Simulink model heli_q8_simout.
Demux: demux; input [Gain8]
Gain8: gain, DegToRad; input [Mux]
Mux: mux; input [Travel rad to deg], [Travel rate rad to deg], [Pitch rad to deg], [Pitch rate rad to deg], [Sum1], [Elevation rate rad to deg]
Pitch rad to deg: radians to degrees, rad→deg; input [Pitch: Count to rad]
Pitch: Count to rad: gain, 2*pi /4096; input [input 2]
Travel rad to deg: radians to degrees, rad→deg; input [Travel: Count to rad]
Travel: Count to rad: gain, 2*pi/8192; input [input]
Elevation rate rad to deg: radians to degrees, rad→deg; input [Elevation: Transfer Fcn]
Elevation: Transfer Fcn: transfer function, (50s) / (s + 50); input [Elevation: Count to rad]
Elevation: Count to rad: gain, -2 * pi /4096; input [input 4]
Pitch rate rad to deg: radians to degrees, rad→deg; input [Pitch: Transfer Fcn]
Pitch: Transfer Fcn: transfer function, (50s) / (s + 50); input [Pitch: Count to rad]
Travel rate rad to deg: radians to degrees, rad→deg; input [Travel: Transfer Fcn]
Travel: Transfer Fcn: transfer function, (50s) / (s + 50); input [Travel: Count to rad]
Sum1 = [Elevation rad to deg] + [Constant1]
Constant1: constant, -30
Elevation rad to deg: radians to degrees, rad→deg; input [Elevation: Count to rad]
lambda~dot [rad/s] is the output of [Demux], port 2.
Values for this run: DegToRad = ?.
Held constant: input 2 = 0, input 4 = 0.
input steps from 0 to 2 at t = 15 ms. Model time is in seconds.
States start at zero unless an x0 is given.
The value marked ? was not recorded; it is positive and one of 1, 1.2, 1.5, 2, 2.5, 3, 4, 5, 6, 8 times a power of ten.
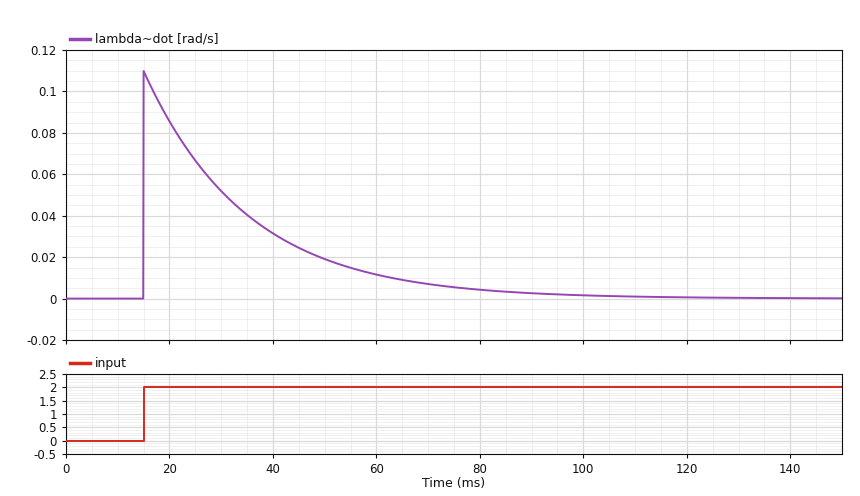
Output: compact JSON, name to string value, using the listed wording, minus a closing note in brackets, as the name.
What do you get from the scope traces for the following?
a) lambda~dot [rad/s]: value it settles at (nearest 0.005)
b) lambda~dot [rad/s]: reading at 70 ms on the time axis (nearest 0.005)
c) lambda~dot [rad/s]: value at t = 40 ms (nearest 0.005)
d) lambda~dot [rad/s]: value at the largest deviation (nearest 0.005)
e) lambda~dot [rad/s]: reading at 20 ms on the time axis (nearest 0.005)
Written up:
{"lambda~dot [rad/s]: value it settles at": "0.000", "lambda~dot [rad/s]: reading at 70 ms on the time axis": "0.005", "lambda~dot [rad/s]: value at t = 40 ms": "0.030", "lambda~dot [rad/s]: value at the largest deviation": "0.110", "lambda~dot [rad/s]: reading at 20 ms on the time axis": "0.085"}
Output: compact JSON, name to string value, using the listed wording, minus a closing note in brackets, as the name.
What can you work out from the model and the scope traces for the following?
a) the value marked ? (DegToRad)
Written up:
{"the value marked ?": "0.025"}
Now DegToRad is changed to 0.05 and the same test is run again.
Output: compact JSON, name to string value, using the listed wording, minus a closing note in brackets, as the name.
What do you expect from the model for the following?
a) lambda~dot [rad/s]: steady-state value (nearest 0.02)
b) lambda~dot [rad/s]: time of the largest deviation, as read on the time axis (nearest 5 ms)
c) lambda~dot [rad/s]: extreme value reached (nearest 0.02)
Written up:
{"lambda~dot [rad/s]: steady-state value": "0.00", "lambda~dot [rad/s]: time of the largest deviation, as read on the time axis": "15 ms", "lambda~dot [rad/s]: extreme value reached": "0.22"}
